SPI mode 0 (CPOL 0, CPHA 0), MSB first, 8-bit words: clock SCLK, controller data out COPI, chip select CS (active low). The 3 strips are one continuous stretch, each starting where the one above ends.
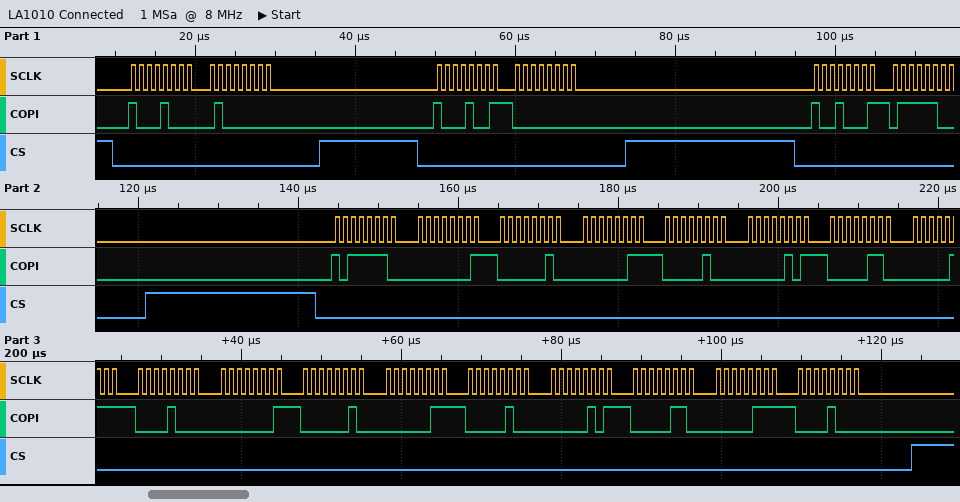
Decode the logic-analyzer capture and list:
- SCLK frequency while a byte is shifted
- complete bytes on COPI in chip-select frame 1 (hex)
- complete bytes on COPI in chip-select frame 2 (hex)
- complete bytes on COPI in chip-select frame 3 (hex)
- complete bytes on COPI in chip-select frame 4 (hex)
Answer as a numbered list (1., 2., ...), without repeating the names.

1. 1 MHz
2. 88 40
3. 89 00
4. 91 7C
5. BE 01 02 03 04 05 06 07 08 01 02 03 04 05 06 07 08
